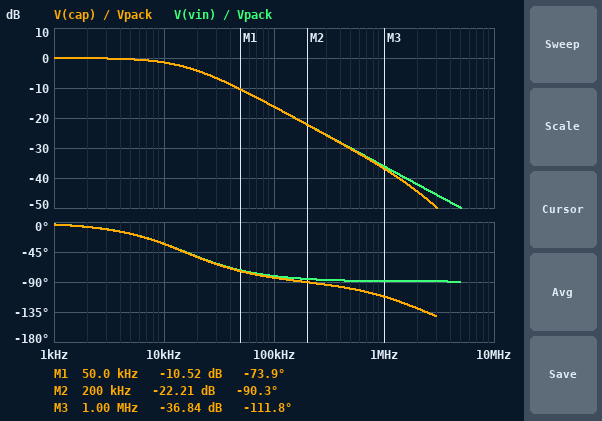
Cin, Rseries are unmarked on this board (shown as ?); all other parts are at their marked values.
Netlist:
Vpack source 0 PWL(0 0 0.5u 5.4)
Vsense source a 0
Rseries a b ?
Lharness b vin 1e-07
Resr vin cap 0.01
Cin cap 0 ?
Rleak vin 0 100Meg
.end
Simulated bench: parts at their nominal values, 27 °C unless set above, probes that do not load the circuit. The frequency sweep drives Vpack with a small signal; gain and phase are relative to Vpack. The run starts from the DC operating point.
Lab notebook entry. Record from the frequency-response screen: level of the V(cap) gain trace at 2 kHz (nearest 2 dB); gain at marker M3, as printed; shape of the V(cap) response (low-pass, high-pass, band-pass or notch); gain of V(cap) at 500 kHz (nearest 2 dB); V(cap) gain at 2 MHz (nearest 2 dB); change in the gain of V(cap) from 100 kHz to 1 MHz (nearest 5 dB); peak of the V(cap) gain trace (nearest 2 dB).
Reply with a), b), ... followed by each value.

a) 0 dB
b) -36.84 dB
c) low-pass
d) -30 dB
e) -44 dB
f) -20 dB
g) 0 dB
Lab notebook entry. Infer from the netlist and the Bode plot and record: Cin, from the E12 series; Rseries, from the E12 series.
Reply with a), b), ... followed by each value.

a) 6.8 µF
b) 1.5 Ω
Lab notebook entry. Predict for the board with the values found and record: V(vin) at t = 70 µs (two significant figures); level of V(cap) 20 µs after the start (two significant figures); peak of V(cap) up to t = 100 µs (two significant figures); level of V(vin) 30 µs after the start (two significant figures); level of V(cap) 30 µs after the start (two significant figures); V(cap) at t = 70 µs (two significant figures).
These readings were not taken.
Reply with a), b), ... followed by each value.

a) 5.4 V
b) 4.6 V
c) 5.4 V
d) 5.1 V
e) 5.1 V
f) 5.4 V
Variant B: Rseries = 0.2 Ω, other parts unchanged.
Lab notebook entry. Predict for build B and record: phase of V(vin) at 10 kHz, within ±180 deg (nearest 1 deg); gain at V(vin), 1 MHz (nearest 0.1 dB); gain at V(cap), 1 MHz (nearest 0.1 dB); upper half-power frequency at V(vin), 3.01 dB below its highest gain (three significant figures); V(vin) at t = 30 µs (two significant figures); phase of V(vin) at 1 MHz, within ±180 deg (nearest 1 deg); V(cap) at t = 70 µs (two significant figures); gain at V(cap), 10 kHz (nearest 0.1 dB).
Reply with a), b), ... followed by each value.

a) -5 deg
b) -28.0 dB
c) -28.7 dB
d) 152 kHz
e) 5.4 V
f) -138 deg
g) 5.4 V
h) 0 dB
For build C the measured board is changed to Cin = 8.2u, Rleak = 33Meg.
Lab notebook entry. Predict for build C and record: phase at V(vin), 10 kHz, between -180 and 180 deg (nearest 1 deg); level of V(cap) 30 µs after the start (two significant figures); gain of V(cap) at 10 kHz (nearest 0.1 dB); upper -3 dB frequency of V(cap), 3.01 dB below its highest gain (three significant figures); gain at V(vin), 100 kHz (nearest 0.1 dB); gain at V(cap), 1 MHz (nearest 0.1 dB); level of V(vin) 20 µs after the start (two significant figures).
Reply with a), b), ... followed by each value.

a) -38 deg
b) 4.9 V
c) -2.0 dB
d) 12.9 kHz
e) -17.8 dB
f) -38.5 dB
g) 4.3 V
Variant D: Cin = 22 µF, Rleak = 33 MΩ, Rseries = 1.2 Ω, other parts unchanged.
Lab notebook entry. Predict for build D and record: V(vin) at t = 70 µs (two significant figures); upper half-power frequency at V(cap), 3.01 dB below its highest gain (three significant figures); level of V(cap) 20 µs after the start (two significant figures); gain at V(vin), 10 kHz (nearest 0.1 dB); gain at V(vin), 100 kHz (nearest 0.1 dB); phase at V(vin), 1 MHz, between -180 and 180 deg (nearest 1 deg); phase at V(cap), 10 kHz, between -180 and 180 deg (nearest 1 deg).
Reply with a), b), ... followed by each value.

a) 5.0 V
b) 6.00 kHz
c) 2.8 V
d) -5.8 dB
e) -24.4 dB
f) -63 deg
g) -59 deg
